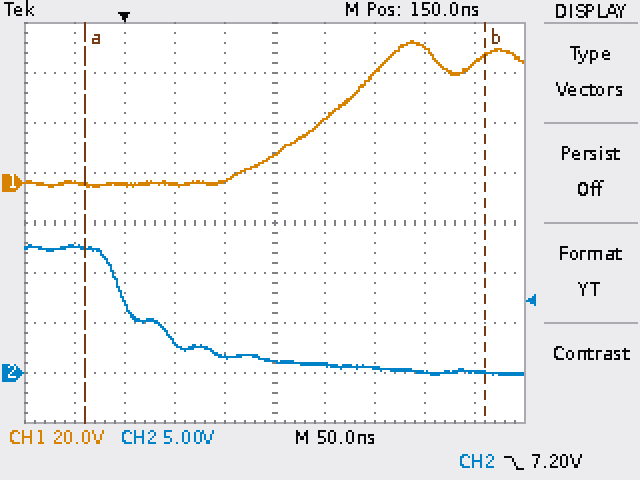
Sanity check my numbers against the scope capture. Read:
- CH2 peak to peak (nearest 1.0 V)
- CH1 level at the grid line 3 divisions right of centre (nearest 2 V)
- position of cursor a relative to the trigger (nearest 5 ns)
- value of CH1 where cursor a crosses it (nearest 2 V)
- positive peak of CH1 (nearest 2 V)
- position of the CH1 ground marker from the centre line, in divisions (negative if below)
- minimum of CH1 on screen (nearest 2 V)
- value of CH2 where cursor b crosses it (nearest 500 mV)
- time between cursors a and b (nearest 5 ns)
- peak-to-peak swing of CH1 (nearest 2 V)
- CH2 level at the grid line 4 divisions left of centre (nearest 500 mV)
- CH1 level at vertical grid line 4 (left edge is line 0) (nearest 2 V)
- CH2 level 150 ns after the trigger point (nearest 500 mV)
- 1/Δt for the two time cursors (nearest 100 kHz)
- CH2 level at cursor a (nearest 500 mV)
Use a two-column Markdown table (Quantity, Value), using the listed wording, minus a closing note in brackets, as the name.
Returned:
| Quantity | Value |
|---|---|
| CH2 peak to peak | 13.0 V |
| CH1 level at the grid line 3 divisions right of centre | 54 V |
| position of cursor a relative to the trigger | -40 ns |
| value of CH1 where cursor a crosses it | 0 V |
| positive peak of CH1 | 56 V |
| position of the CH1 ground marker from the centre line, in divisions | +0.8 div |
| minimum of CH1 on screen | -2 V |
| value of CH2 where cursor b crosses it | 0.0 V |
| time between cursors a and b | 400 ns |
| peak-to-peak swing of CH1 | 58 V |
| CH2 level at the grid line 4 divisions left of centre | 12.5 V |
| CH1 level at vertical grid line 4 (left edge is line 0) | 0 V |
| CH2 level 150 ns after the trigger point | 1.0 V |
| 1/Δt for the two time cursors | 2.5 MHz |
| CH2 level at cursor a | 12.5 V |
